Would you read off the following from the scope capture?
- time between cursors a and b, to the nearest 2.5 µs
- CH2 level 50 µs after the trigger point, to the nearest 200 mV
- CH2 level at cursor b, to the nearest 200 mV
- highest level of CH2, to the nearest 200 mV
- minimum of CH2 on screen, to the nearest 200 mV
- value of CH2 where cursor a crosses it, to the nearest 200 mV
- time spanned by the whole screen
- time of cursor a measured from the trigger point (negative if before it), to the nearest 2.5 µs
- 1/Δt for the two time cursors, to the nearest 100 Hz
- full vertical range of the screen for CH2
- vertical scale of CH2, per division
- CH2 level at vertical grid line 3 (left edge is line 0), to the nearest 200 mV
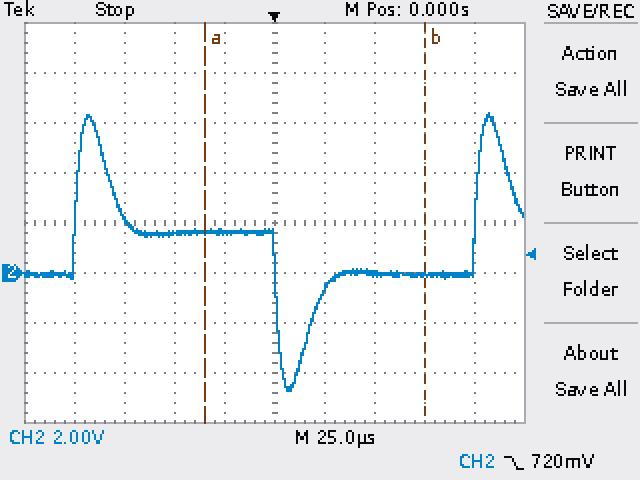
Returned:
110.0 µs
0.0 V
0.0 V
6.4 V
-4.8 V
1.6 V
250 µs
-35.0 µs
9.1 kHz
16 V
2 V
1.6 V
